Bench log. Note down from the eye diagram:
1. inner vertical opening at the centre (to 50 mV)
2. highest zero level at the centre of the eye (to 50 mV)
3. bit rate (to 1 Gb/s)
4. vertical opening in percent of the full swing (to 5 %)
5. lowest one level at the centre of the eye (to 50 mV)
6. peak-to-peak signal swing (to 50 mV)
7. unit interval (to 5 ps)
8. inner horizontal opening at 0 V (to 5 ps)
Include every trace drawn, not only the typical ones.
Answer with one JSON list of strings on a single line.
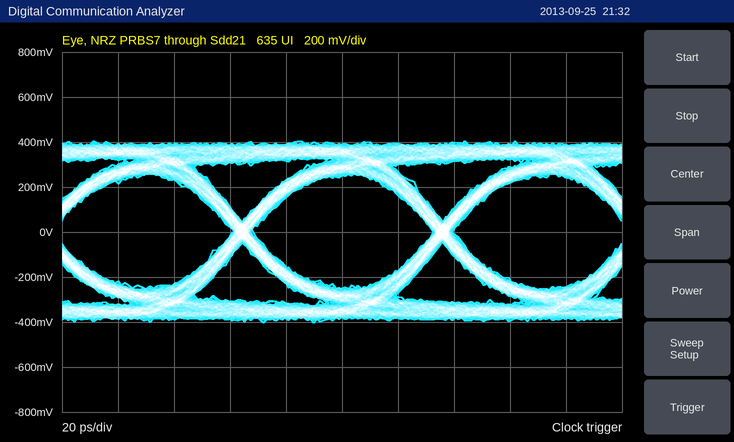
["500 mV", "-250 mV", "14 Gb/s", "60 %", "250 mV", "800 mV", "70 ps", "65 ps"]
